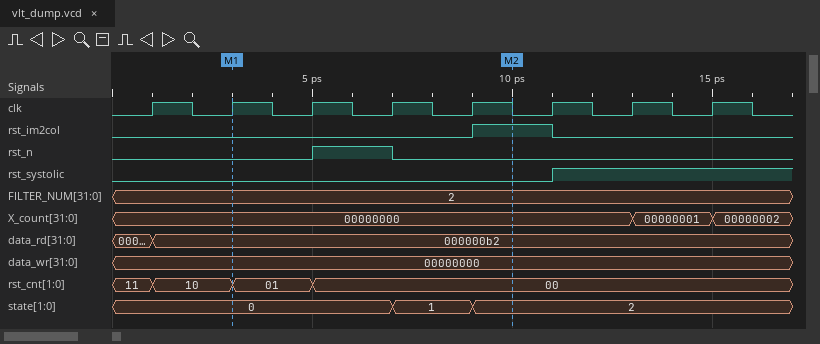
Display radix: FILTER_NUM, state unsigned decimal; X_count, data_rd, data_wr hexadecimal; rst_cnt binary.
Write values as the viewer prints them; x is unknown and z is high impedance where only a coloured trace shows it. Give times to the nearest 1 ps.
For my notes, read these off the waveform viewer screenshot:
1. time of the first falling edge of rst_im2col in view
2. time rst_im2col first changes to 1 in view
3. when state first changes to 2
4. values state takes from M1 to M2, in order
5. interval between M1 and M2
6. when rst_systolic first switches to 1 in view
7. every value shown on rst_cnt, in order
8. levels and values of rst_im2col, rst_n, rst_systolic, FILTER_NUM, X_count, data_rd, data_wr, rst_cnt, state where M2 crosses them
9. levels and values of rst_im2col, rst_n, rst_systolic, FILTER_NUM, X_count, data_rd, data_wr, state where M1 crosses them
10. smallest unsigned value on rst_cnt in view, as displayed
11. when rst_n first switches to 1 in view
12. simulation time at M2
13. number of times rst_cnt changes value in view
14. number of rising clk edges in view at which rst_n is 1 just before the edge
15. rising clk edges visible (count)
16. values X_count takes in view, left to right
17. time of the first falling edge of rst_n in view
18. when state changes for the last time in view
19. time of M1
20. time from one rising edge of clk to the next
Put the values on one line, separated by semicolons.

11 ps; 9 ps; 9 ps; 0, 1, 2; 7 ps; 11 ps; 11, 10, 01, 00; rst_im2col=1, rst_n=0, rst_systolic=0, FILTER_NUM=2, X_count=00000000, data_rd=000000b2, data_wr=00000000, rst_cnt=00, state=2; rst_im2col=0, rst_n=0, rst_systolic=0, FILTER_NUM=2, X_count=00000000, data_rd=000000b2, data_wr=00000000, state=0; 00; 5 ps; 10 ps; 3; 1; 8; 00000000, 00000001, 00000002; 7 ps; 9 ps; 3 ps; 2 ps
